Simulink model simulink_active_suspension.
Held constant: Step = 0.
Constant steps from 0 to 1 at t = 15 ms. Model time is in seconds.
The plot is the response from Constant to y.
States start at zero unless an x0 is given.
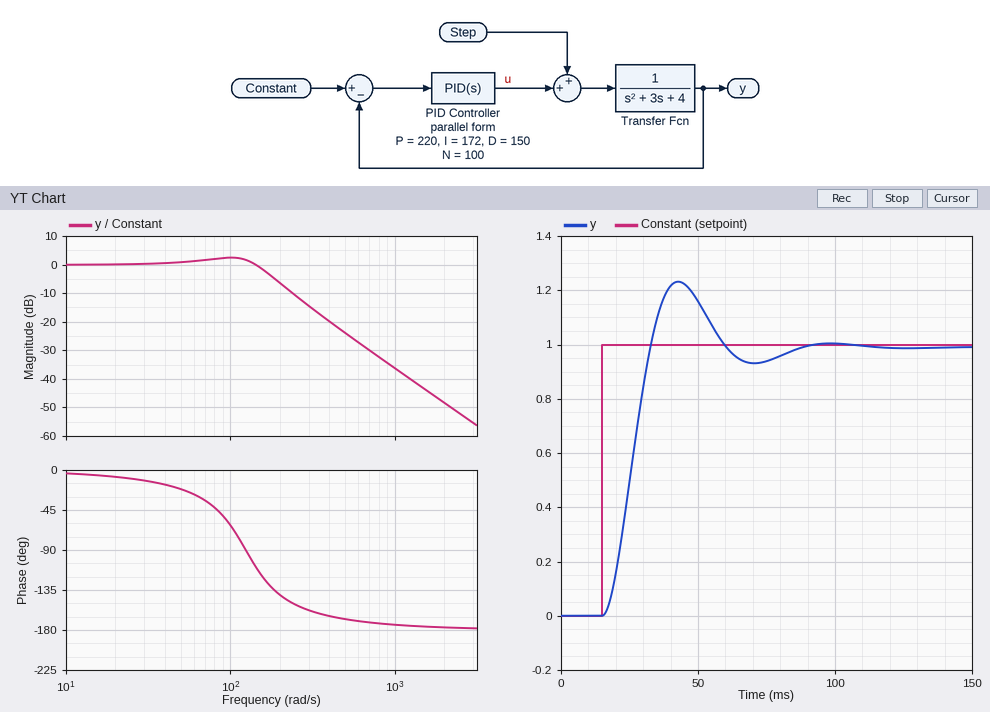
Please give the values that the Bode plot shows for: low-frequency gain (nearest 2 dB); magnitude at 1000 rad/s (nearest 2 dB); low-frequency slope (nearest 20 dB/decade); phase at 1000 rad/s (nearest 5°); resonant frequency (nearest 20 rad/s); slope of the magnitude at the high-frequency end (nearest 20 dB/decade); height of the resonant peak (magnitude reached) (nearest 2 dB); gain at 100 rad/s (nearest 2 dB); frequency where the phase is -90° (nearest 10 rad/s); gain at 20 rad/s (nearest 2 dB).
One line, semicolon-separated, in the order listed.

0 dB; -36 dB; 0 dB/decade; -175°; 100 rad/s; -40 dB/decade; 2 dB; 2 dB; 120 rad/s; 0 dB
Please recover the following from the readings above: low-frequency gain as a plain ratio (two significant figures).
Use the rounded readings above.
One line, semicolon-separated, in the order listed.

1.0
